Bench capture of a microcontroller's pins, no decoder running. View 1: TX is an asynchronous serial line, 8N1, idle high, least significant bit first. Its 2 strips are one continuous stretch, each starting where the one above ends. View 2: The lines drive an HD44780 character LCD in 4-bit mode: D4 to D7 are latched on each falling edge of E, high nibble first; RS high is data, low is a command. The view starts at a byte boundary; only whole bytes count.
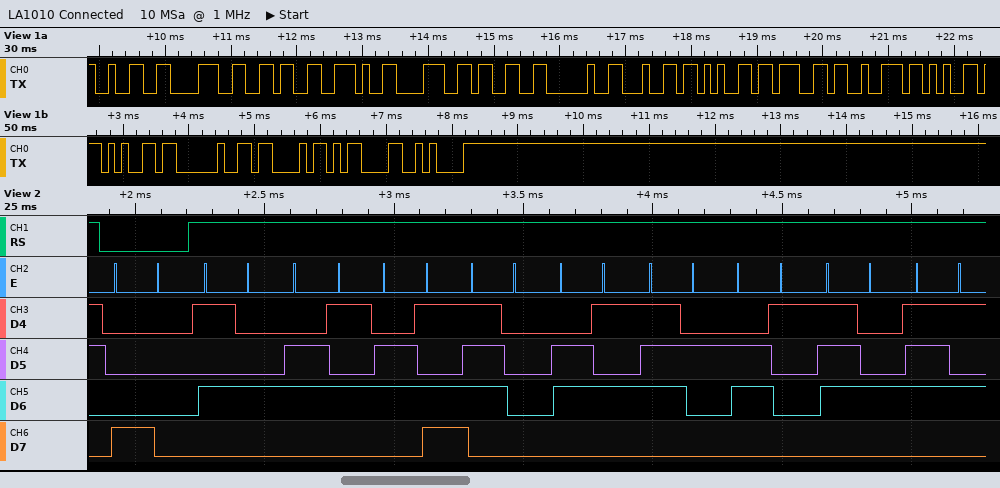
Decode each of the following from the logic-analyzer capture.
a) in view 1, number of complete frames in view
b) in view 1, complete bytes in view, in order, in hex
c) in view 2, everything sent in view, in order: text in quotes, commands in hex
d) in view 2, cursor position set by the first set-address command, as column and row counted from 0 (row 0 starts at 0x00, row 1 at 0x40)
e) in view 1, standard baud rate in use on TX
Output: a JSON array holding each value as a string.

["17", "0x32 0x38 0x36 0x2E 0x38 0x33 0x20 0x64 0x65 0x67 0x72 0x65 0x65 0x20 0x43 0x0D 0x0A", "0x80 \"Temperatu\"", "column 0, row 0", "9600 baud"]
